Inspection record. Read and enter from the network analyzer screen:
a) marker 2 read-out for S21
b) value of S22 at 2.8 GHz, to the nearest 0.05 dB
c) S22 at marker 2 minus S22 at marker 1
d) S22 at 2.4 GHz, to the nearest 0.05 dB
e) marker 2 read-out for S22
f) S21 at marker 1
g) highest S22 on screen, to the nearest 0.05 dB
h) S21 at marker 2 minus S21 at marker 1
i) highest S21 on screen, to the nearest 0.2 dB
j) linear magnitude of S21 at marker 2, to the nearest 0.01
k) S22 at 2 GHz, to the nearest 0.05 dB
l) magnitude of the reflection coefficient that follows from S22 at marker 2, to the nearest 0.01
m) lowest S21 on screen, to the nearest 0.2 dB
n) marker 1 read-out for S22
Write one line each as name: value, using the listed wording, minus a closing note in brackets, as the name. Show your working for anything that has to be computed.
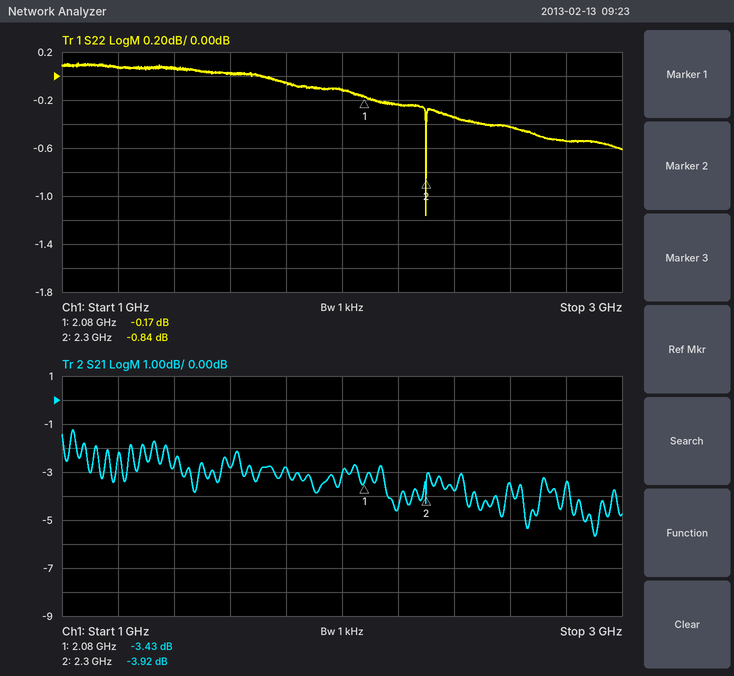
marker 2 read-out for S21: -3.92 dB
value of S22 at 2.8 GHz, to the nearest 0.05 dB: -0.55 dB
S22 at marker 2 minus S22 at marker 1: -0.84 − (-0.17) = -0.67 dB
S22 at 2.4 GHz, to the nearest 0.05 dB: -0.35 dB
marker 2 read-out for S22: -0.84 dB
S21 at marker 1: -3.43 dB
highest S22 on screen, to the nearest 0.05 dB: 0.10 dB
S21 at marker 2 minus S21 at marker 1: -3.92 − (-3.43) = -0.49 dB
highest S21 on screen, to the nearest 0.2 dB: -1.2 dB
linear magnitude of S21 at marker 2, to the nearest 0.01: 10^(-3.92/20) ≈ 0.64
S22 at 2 GHz, to the nearest 0.05 dB: -0.10 dB
magnitude of the reflection coefficient that follows from S22 at marker 2, to the nearest 0.01: 10^(-0.84/20) ≈ 0.91
lowest S21 on screen, to the nearest 0.2 dB: -5.6 dB
marker 1 read-out for S22: -0.17 dB
